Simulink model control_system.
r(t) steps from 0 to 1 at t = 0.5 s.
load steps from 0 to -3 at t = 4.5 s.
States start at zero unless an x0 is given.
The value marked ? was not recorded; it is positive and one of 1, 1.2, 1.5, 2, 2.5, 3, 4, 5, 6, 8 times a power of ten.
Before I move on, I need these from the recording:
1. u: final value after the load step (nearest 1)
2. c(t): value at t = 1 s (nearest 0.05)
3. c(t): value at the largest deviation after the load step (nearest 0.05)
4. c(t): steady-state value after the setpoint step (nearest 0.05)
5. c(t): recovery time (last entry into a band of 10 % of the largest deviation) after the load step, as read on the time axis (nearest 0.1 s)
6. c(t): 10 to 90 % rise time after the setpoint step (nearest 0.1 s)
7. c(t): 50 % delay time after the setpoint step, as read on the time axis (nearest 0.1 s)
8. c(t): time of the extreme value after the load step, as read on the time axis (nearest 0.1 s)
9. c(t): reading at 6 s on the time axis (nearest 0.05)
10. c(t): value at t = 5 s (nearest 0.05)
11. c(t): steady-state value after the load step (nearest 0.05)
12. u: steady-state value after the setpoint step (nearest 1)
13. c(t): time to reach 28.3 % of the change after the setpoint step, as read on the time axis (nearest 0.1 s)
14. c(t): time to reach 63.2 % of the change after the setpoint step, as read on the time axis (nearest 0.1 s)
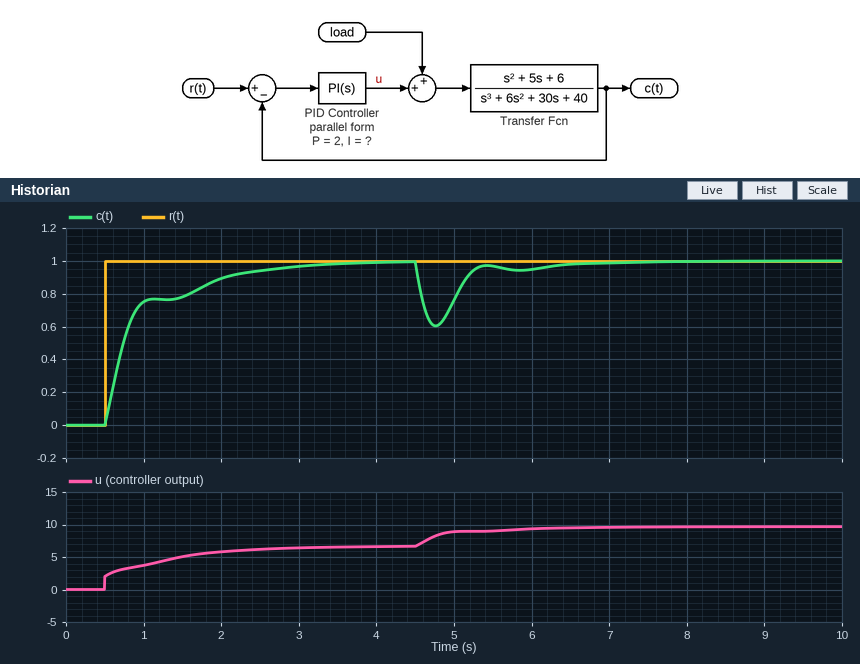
10
0.75
0.60
1.00
6.2 s
1.5 s
0.7 s
4.8 s
0.95
0.75
1.00
7
0.6 s
0.8 s
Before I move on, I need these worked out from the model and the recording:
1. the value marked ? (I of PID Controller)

12
